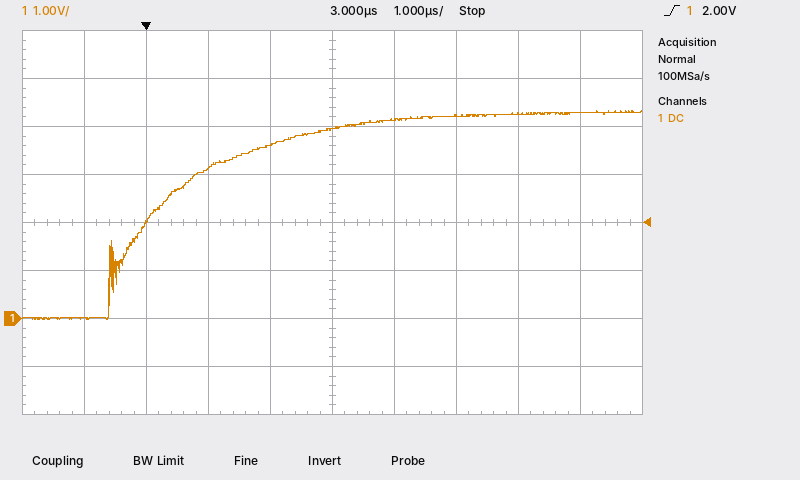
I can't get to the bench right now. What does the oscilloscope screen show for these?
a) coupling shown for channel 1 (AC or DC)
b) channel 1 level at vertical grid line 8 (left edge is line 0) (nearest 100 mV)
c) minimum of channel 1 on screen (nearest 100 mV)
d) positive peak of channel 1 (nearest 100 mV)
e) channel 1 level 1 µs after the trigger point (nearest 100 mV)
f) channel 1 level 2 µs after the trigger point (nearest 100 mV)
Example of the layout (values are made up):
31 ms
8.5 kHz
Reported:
DC
4.3 V
0.0 V
4.3 V
3.1 V
3.6 V
